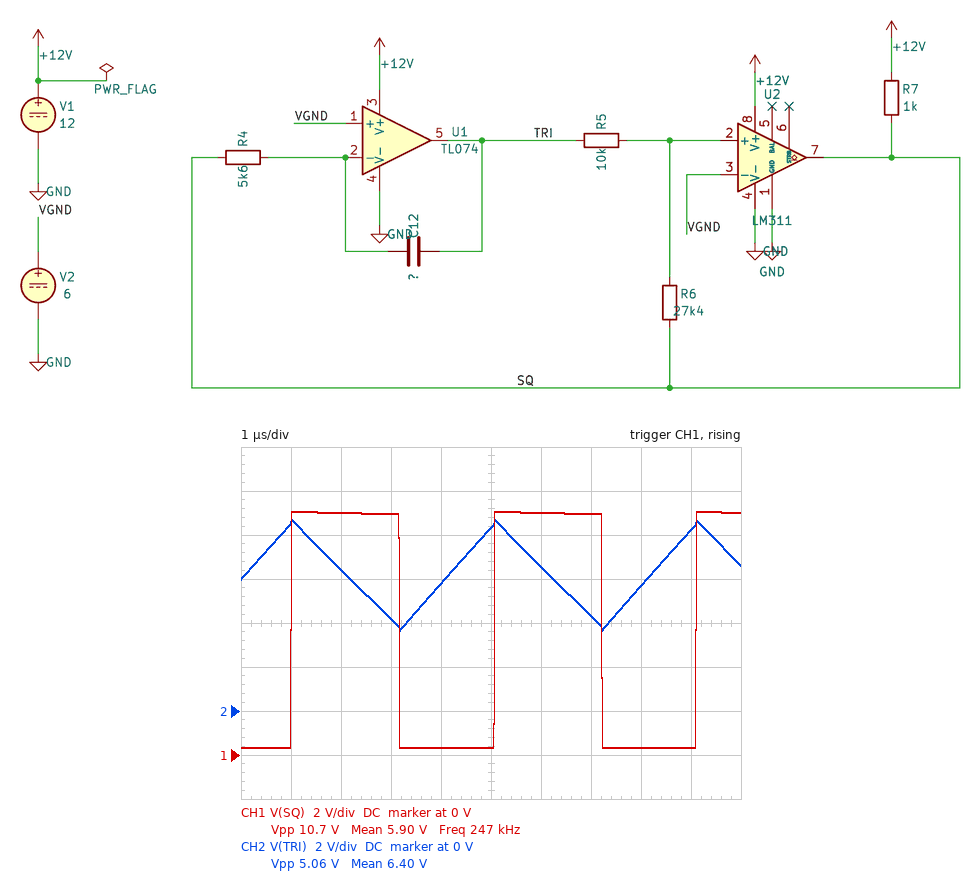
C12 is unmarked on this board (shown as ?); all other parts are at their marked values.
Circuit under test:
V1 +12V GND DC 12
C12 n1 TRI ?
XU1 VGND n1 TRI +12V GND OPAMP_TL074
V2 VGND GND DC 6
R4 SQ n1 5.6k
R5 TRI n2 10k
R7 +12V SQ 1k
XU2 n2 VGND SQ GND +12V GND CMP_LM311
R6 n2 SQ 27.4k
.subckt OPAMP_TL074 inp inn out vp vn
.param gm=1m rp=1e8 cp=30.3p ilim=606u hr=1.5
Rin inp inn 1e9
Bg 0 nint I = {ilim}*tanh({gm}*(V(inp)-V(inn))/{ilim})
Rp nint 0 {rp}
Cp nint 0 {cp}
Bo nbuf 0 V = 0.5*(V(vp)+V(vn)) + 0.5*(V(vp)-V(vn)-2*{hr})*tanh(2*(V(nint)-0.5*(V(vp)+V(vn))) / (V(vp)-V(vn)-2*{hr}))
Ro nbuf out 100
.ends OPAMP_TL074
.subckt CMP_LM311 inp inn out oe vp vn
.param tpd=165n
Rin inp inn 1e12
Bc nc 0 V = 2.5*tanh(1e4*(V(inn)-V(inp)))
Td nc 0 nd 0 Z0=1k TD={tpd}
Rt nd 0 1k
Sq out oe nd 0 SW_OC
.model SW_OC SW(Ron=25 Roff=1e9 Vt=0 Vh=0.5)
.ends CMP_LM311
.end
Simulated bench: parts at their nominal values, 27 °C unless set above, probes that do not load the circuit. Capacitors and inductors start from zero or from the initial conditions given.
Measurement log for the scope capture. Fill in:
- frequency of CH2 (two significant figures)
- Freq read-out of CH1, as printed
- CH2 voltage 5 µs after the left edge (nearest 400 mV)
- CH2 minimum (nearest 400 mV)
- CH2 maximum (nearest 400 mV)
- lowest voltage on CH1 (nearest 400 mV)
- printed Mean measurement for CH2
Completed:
250 kHz
247 kHz
8.4 V
3.6 V
8.8 V
400 mV
6.40 V
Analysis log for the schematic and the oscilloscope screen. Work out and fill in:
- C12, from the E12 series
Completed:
390 pF
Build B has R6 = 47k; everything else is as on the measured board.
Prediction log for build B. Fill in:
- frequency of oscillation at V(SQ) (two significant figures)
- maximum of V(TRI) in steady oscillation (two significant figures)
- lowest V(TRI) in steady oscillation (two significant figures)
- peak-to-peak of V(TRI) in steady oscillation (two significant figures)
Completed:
370 kHz
7.8 V
4.4 V
3.5 V
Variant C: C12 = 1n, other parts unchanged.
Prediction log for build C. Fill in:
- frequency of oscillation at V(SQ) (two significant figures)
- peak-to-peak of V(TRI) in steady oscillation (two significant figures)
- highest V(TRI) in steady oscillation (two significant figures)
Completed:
110 kHz
4.6 V
8.4 V
